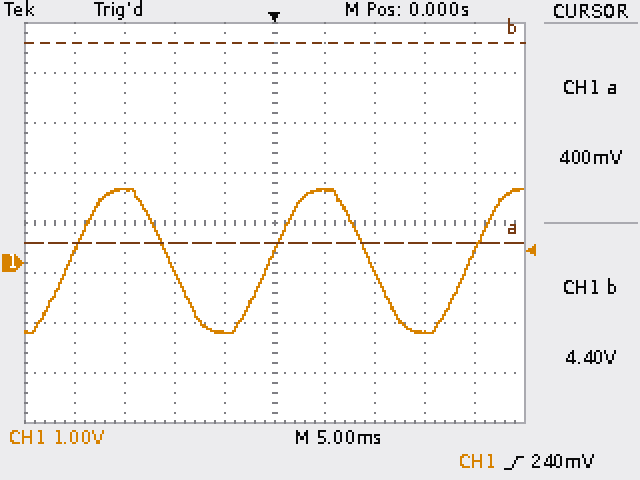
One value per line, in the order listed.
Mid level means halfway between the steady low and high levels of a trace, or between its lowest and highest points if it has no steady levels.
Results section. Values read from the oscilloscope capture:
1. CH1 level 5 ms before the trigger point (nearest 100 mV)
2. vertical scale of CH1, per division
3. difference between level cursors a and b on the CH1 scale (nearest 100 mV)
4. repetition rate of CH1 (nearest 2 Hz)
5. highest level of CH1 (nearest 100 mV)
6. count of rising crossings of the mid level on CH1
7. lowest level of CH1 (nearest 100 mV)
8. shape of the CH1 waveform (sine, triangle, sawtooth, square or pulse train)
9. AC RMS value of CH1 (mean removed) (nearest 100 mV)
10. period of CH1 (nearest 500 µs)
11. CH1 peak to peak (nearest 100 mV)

-1.4 V
1 V
4.0 V
50 Hz
1.5 V
3
-1.4 V
sine
1.0 V
20.0 ms
2.9 V
